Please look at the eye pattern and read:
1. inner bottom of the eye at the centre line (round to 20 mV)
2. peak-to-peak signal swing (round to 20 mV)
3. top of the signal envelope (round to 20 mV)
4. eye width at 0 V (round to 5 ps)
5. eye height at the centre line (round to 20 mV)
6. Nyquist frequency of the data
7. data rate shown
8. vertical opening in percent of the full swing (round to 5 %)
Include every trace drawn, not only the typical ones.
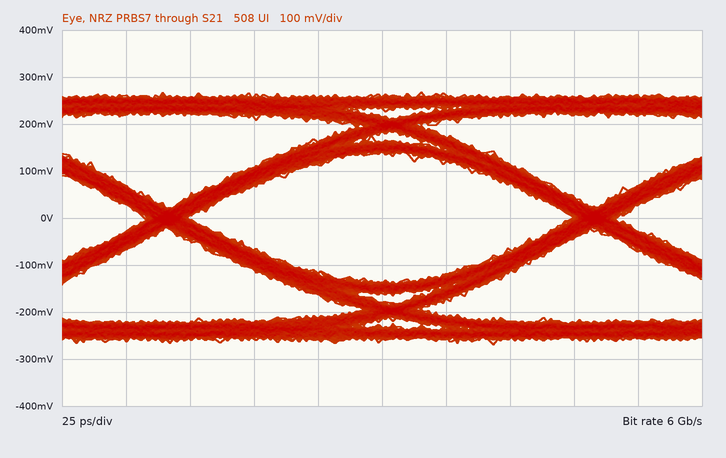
-140 mV
540 mV
260 mV
150 ps
280 mV
3 GHz
6 Gb/s
50 %
